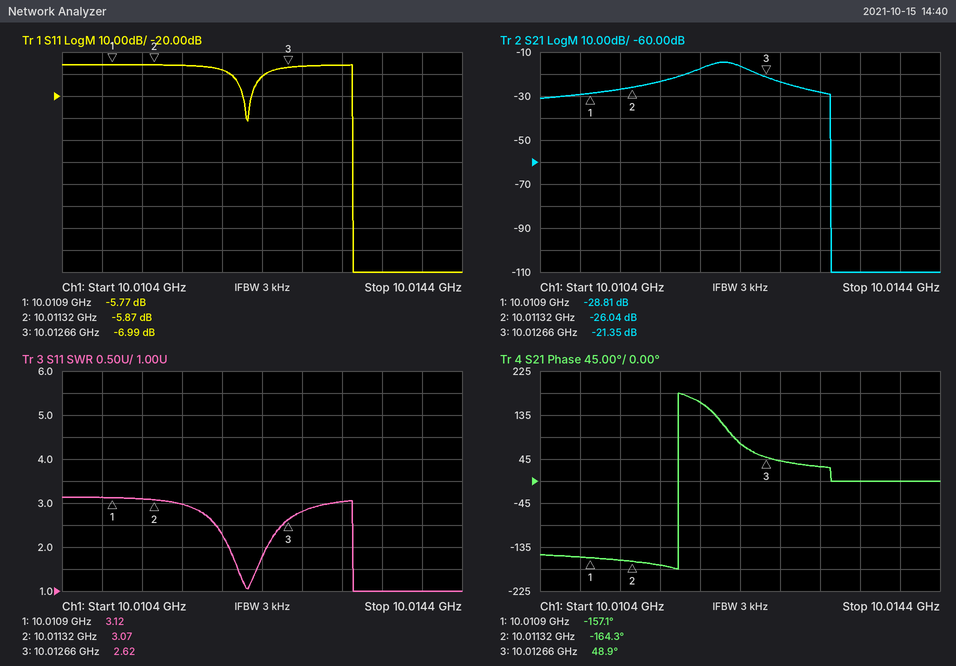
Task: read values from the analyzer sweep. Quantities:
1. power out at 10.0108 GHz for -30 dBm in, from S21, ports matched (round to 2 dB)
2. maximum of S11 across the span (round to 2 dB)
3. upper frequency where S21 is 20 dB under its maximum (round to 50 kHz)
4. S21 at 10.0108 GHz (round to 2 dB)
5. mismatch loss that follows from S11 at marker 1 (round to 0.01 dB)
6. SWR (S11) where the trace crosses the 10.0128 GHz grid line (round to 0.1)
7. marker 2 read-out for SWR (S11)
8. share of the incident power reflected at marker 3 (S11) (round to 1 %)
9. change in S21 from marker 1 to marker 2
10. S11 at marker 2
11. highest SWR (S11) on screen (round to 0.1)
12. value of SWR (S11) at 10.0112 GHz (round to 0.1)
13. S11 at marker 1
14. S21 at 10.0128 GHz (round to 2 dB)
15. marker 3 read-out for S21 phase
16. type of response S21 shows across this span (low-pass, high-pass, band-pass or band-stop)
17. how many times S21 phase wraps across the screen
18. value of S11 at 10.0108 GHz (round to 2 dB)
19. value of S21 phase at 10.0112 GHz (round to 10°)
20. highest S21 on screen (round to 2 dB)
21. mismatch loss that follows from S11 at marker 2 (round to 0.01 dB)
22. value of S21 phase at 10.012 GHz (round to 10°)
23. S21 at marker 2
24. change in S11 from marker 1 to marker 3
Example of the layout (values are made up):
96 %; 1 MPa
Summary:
-60 dBm; -6 dB; 10.01330 GHz; -30 dB; 1.34 dB; 2.8; 3.07; 20 %; 2.77 dB; -5.87 dB; 3.1; 3.1; -5.77 dB; -24 dB; 48.9°; band-pass; 1; -6 dB; -160°; -14 dB; 1.30 dB; 160°; -26.04 dB; -1.22 dB
